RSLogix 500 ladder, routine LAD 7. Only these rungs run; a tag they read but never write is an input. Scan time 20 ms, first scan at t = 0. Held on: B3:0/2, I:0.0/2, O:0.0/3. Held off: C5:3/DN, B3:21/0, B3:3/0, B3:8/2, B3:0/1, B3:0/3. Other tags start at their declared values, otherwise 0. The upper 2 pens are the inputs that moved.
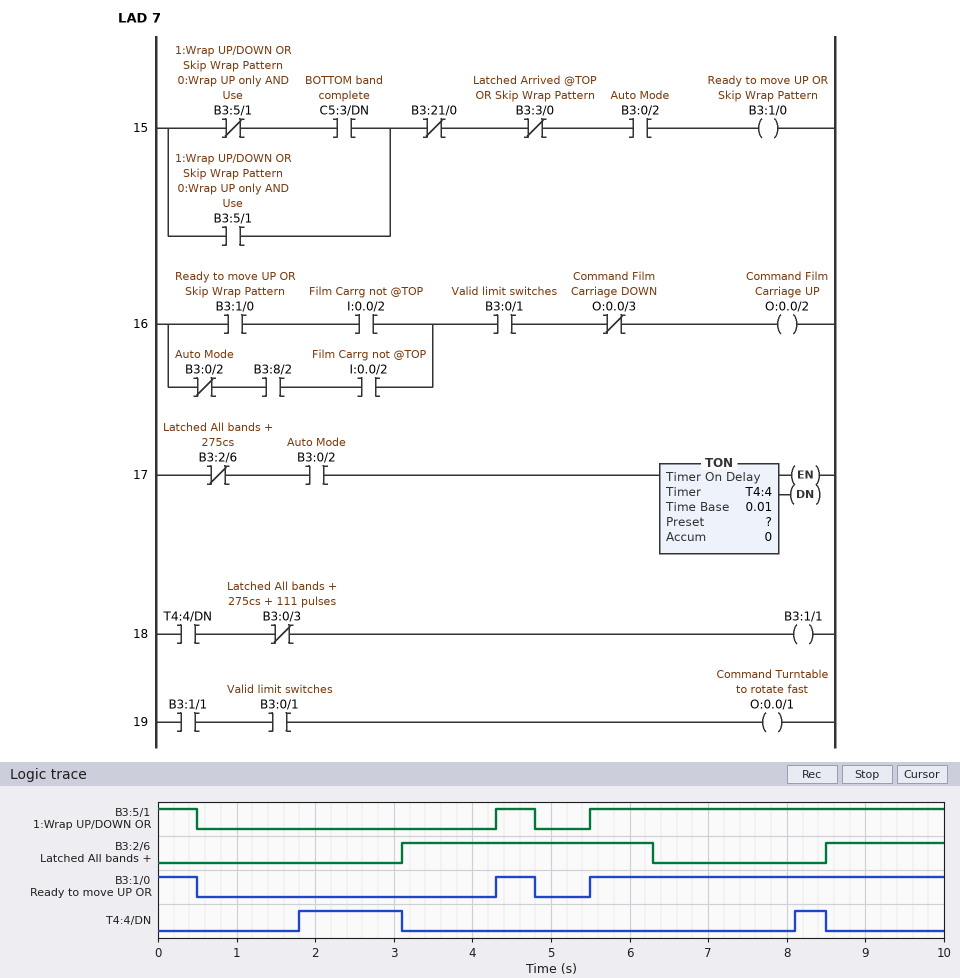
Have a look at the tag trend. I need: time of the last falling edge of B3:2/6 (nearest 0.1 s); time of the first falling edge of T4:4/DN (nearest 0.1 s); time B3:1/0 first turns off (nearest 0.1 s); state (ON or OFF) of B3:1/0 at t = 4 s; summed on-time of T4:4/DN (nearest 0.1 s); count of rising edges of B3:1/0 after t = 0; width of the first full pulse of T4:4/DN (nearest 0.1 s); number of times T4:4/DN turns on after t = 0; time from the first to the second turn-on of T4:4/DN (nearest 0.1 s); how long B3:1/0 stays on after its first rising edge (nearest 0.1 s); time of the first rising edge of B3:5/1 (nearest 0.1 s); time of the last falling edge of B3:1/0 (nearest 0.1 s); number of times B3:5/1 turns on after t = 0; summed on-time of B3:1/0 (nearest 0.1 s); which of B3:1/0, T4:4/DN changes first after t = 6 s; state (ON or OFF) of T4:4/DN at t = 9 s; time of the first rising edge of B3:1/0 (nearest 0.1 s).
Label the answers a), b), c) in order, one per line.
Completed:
a) 6.3 s
b) 3.1 s
c) 0.5 s
d) OFF
e) 1.7 s
f) 2
g) 1.3 s
h) 2
i) 6.3 s
j) 0.5 s
k) 4.3 s
l) 4.8 s
m) 2
n) 5.5 s
o) T4:4/DN
p) OFF
q) 4.3 s
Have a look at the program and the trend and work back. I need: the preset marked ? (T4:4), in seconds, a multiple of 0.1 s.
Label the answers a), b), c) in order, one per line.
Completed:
a) 1.8 s
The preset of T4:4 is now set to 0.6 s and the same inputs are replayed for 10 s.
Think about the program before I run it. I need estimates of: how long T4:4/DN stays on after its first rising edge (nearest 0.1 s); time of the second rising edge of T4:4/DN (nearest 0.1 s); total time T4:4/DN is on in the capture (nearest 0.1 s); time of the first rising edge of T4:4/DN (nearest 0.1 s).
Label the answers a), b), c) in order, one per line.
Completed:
a) 2.5 s
b) 6.9 s
c) 4.1 s
d) 0.6 s
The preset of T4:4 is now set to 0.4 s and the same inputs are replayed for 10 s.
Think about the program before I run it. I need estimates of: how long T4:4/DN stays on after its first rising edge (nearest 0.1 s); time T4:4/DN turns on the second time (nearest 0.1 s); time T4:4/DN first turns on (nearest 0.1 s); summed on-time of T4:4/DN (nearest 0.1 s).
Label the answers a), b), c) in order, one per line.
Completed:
a) 2.7 s
b) 6.7 s
c) 0.4 s
d) 4.5 s
